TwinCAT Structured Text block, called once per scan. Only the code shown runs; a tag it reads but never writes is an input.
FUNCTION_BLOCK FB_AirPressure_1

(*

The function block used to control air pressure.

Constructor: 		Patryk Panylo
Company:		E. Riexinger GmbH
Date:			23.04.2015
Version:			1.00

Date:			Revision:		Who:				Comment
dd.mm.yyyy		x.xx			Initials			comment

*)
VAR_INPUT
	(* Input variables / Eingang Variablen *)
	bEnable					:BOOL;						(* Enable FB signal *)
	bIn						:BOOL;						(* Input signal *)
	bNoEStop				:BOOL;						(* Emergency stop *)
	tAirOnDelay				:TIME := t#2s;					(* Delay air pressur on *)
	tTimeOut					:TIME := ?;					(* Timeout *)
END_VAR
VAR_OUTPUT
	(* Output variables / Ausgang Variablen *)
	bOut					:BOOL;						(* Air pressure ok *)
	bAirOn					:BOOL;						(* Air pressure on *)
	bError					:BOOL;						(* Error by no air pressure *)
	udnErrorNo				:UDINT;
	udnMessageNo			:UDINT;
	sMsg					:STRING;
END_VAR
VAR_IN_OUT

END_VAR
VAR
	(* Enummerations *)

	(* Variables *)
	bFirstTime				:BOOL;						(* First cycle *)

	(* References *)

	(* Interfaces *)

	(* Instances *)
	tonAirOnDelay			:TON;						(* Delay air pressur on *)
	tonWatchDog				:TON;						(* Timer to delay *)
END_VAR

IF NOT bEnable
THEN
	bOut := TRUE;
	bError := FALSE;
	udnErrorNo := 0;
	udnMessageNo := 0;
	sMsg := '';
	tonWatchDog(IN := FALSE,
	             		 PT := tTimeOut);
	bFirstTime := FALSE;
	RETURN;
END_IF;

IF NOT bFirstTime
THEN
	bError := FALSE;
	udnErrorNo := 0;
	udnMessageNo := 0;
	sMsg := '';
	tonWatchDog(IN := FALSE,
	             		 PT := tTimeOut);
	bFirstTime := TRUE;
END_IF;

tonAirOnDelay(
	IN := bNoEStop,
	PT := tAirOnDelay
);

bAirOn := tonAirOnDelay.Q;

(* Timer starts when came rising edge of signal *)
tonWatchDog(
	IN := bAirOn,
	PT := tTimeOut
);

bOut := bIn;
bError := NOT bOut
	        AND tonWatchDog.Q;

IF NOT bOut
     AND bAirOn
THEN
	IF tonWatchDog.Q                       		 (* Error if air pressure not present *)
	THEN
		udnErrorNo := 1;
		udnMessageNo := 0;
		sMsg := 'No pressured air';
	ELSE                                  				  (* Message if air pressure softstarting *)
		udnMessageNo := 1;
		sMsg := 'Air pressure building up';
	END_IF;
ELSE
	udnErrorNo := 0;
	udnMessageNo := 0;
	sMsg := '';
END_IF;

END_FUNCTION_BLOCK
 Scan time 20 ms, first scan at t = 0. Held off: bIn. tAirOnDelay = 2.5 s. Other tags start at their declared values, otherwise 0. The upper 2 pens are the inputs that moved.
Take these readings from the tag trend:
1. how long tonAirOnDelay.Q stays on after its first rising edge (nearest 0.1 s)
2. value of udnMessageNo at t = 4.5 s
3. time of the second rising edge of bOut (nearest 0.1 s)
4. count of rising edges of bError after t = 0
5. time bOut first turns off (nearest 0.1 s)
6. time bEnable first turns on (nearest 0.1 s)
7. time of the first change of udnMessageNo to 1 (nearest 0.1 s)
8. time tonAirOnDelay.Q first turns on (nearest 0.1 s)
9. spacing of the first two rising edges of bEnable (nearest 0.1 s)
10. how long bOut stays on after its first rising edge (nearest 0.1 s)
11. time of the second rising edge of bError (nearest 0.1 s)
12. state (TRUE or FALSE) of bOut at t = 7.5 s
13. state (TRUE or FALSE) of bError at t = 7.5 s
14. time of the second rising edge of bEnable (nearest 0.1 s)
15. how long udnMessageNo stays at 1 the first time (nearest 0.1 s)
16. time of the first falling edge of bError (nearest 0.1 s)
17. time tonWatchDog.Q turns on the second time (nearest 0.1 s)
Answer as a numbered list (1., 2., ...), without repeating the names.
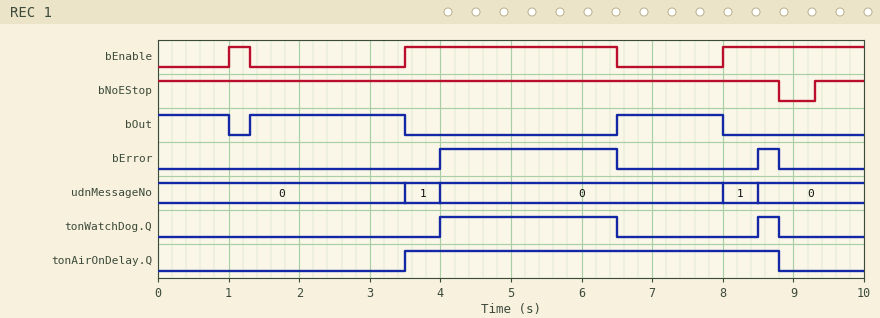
1. 5.3 s
2. 0
3. 6.5 s
4. 2
5. 1.0 s
6. 1.0 s
7. 3.5 s
8. 3.5 s
9. 2.5 s
10. 2.2 s
11. 8.5 s
12. TRUE
13. FALSE
14. 3.5 s
15. 0.5 s
16. 6.5 s
17. 8.5 s
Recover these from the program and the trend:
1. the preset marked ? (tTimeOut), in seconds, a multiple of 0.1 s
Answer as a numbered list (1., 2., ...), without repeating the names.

1. 0.5 s
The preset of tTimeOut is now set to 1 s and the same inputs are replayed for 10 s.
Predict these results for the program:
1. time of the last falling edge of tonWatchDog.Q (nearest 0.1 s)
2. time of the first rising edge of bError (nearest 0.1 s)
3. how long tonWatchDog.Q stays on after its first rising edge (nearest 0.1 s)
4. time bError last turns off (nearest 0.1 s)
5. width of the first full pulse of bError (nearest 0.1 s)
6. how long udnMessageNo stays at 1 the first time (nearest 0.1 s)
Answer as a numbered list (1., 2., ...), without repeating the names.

1. 6.5 s
2. 4.5 s
3. 2.0 s
4. 6.5 s
5. 2.0 s
6. 1.0 s
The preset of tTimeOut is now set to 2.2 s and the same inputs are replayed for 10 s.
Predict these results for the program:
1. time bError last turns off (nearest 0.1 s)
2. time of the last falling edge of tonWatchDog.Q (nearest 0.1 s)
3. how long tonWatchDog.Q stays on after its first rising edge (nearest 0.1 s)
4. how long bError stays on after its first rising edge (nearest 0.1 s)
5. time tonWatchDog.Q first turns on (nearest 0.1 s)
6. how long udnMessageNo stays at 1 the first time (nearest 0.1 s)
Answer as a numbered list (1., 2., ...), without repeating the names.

1. 6.5 s
2. 6.5 s
3. 0.8 s
4. 0.8 s
5. 5.7 s
6. 2.2 s
